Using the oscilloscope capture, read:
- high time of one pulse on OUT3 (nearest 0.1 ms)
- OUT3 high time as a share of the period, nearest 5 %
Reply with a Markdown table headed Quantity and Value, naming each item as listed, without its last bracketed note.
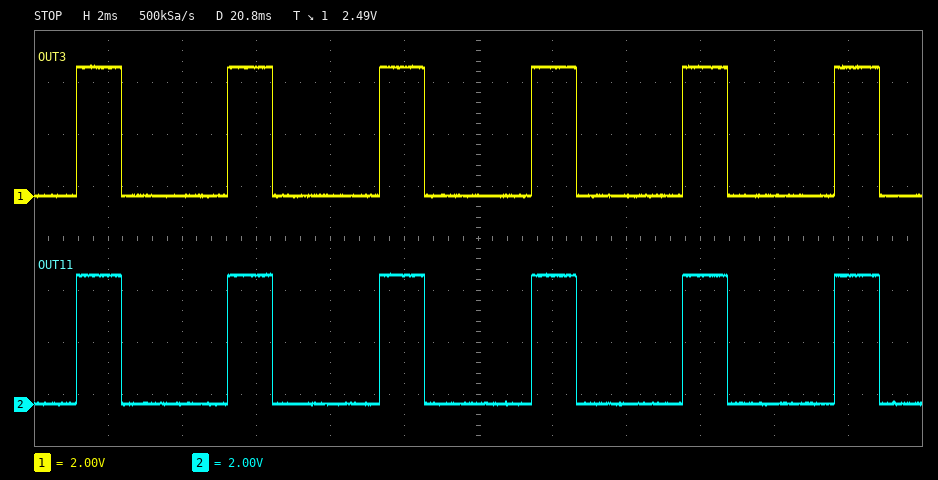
| Quantity | Value |
|---|---|
| high time of one pulse on OUT3 | 1.2 ms |
| OUT3 high time as a share of the period, nearest 5 % | 30 % |
